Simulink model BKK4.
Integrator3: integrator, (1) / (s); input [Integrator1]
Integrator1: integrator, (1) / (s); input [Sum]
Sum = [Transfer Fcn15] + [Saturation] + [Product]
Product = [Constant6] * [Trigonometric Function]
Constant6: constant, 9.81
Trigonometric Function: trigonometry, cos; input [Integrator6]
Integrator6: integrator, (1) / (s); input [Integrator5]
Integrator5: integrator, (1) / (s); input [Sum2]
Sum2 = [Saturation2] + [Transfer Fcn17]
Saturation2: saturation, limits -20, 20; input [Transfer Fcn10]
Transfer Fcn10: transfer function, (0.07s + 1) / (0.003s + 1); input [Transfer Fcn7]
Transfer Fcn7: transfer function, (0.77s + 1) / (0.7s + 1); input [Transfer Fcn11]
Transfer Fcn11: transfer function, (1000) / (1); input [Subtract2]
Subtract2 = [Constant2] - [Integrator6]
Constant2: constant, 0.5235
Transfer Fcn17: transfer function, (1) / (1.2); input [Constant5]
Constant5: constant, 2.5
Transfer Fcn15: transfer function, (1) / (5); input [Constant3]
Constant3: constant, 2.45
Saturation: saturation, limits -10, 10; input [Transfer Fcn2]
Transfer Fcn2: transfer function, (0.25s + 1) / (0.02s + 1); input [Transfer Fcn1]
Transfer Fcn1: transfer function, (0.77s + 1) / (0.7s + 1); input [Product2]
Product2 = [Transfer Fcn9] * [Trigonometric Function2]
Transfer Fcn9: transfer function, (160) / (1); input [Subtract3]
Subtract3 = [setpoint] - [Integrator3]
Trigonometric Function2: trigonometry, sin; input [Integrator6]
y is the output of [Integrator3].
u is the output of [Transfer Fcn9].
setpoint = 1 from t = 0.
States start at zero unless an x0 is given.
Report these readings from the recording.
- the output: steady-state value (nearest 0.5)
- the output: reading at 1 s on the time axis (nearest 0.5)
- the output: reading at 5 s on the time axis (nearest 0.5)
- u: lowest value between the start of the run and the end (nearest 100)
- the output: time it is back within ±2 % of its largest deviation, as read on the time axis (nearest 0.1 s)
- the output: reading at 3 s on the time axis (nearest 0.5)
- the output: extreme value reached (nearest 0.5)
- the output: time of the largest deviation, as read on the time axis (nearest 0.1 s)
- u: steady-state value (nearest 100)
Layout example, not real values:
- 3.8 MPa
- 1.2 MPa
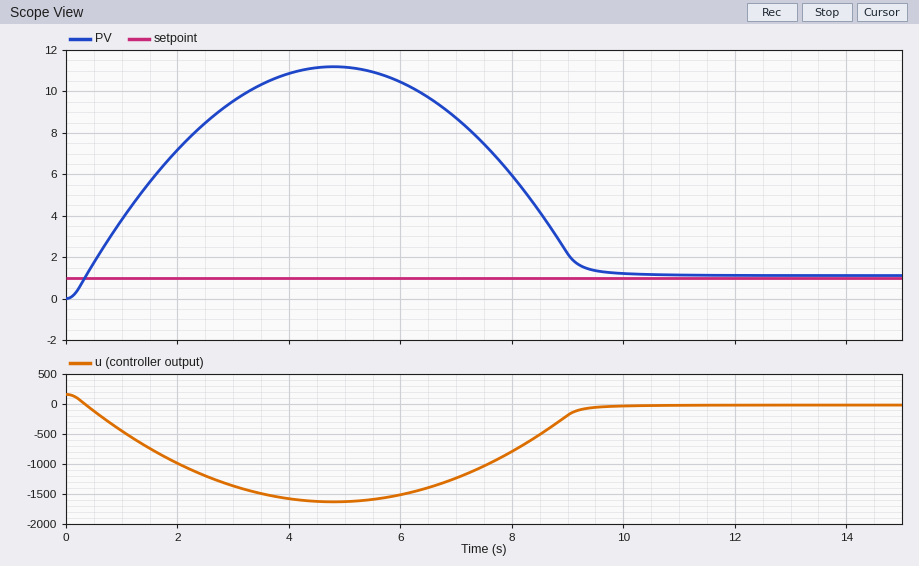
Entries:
- 1.0
- 4.0
- 11.0
- -1600
- 9.5 s
- 9.5
- 11.0
- 4.8 s
- 0
